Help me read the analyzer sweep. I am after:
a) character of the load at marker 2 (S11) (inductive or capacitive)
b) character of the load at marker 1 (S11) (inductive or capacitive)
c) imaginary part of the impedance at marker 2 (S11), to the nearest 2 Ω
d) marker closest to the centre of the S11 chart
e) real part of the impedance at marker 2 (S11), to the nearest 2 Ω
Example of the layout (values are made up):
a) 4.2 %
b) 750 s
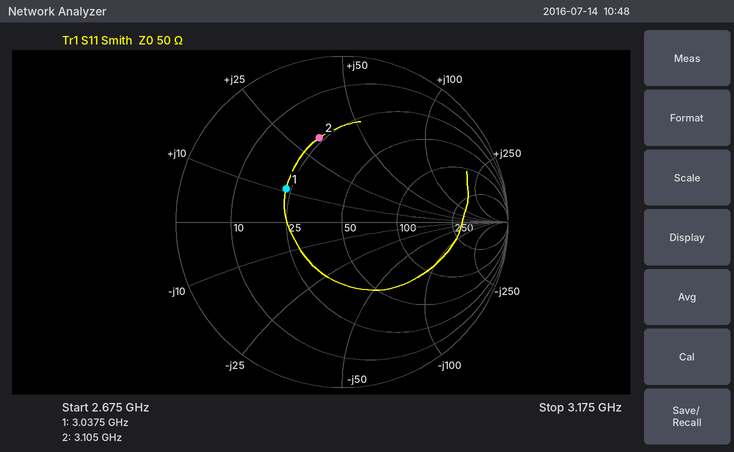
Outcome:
a) inductive
b) inductive
c) +32 Ω
d) marker 1
e) 24 Ω
